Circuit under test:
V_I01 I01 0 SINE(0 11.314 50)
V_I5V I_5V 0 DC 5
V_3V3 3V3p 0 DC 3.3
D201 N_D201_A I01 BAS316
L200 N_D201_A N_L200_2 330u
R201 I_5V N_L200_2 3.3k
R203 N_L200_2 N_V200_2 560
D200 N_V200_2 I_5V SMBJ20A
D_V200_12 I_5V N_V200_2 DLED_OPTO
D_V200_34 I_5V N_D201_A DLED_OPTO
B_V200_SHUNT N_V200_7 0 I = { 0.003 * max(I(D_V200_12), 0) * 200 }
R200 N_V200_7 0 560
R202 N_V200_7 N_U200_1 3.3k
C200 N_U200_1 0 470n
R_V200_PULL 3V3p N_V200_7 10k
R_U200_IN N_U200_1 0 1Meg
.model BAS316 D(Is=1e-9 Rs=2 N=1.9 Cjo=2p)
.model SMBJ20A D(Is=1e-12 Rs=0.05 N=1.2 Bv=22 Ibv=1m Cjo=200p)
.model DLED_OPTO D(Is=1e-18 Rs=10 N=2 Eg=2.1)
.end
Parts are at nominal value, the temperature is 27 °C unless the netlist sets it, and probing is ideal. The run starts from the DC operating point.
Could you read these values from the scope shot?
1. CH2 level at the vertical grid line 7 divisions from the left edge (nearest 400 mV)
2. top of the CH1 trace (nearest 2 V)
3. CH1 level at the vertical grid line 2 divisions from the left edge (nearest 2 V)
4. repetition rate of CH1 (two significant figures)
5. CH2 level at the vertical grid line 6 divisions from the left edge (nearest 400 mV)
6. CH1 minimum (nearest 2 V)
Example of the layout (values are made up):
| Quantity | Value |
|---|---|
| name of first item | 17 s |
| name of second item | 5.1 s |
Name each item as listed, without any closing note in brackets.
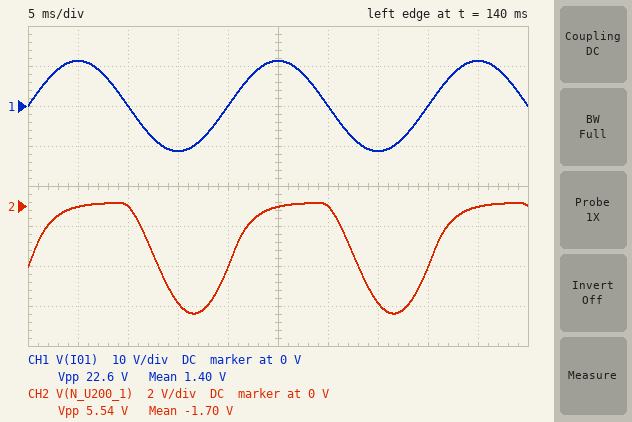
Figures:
| Quantity | Value |
|---|---|
| CH2 level at the vertical grid line 7 divisions from the left edge | -4.8 V |
| top of the CH1 trace | 12 V |
| CH1 level at the vertical grid line 2 divisions from the left edge | 0 V |
| repetition rate of CH1 | 50 Hz |
| CH2 level at the vertical grid line 6 divisions from the left edge | 0 V |
| CH1 minimum | -12 V |
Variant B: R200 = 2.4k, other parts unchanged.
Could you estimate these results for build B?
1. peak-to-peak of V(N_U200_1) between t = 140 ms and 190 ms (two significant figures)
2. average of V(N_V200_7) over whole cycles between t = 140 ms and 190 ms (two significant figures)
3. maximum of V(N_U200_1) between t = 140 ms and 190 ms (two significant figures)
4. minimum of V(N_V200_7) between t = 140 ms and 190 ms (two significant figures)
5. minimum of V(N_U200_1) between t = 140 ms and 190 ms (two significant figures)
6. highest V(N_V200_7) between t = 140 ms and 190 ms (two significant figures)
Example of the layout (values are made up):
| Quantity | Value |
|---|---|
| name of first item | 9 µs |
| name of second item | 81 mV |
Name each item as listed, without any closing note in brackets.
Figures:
| Quantity | Value |
|---|---|
| peak-to-peak of V(N_U200_1) between t = 140 ms and 190 ms | 19 V |
| average of V(N_V200_7) over whole cycles between t = 140 ms and 190 ms | -7.4 V |
| maximum of V(N_U200_1) between t = 140 ms and 190 ms | 330 mV |
| minimum of V(N_V200_7) between t = 140 ms and 190 ms | -20 V |
| minimum of V(N_U200_1) between t = 140 ms and 190 ms | -18 V |
| highest V(N_V200_7) between t = 140 ms and 190 ms | 520 mV |
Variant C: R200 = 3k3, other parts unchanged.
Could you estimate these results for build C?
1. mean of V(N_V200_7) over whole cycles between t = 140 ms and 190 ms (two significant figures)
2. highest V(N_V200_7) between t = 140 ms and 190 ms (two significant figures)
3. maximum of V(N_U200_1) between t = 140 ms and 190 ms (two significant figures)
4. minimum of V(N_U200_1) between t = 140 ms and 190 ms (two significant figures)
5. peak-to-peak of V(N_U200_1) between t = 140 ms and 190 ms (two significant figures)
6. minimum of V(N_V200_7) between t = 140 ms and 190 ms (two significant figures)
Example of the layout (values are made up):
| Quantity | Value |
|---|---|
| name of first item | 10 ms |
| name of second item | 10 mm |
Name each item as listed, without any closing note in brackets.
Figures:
| Quantity | Value |
|---|---|
| mean of V(N_V200_7) over whole cycles between t = 140 ms and 190 ms | -9.4 V |
| highest V(N_V200_7) between t = 140 ms and 190 ms | 560 mV |
| maximum of V(N_U200_1) between t = 140 ms and 190 ms | 250 mV |
| minimum of V(N_U200_1) between t = 140 ms and 190 ms | -23 V |
| peak-to-peak of V(N_U200_1) between t = 140 ms and 190 ms | 23 V |
| minimum of V(N_V200_7) between t = 140 ms and 190 ms | -25 V |
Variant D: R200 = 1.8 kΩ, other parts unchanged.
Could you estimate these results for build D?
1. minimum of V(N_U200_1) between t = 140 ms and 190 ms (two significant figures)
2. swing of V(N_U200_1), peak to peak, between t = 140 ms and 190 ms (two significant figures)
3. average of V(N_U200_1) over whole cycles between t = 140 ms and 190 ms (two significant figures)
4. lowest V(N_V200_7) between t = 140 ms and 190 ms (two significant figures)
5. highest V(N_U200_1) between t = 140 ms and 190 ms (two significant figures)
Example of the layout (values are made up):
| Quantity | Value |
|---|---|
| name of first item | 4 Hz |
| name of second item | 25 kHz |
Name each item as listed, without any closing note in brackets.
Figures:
| Quantity | Value |
|---|---|
| minimum of V(N_U200_1) between t = 140 ms and 190 ms | -15 V |
| swing of V(N_U200_1), peak to peak, between t = 140 ms and 190 ms | 15 V |
| average of V(N_U200_1) over whole cycles between t = 140 ms and 190 ms | -5.8 V |
| lowest V(N_V200_7) between t = 140 ms and 190 ms | -16 V |
| highest V(N_U200_1) between t = 140 ms and 190 ms | 330 mV |
